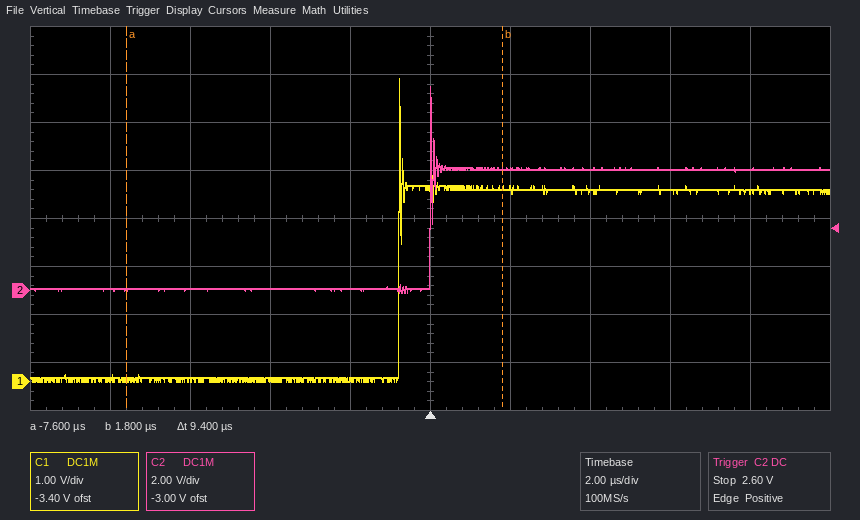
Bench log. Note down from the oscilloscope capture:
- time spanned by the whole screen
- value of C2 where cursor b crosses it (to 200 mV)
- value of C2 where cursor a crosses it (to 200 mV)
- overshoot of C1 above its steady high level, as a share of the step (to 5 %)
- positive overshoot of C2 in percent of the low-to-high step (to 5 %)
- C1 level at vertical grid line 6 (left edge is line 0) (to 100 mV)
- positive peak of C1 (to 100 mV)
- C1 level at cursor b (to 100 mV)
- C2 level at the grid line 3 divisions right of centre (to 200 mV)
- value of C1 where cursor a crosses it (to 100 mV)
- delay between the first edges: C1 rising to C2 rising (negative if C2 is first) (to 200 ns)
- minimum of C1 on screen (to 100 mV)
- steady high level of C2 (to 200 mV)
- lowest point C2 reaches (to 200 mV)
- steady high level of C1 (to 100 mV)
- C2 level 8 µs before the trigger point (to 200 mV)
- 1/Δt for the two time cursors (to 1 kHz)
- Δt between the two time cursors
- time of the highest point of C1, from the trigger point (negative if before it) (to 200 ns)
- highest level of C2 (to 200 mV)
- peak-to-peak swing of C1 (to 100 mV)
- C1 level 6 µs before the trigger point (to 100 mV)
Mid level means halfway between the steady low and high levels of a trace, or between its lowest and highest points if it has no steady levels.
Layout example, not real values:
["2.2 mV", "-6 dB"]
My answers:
["20 µs", "5.0 V", "0.0 V", "60 %", "70 %", "4.0 V", "6.3 V", "4.0 V", "5.0 V", "0.0 V", "+800 ns", "0.0 V", "5.0 V", "0.0 V", "4.0 V", "0.0 V", "106 kHz", "9.4 µs", "-800 ns", "8.4 V", "6.3 V", "0.0 V"]
